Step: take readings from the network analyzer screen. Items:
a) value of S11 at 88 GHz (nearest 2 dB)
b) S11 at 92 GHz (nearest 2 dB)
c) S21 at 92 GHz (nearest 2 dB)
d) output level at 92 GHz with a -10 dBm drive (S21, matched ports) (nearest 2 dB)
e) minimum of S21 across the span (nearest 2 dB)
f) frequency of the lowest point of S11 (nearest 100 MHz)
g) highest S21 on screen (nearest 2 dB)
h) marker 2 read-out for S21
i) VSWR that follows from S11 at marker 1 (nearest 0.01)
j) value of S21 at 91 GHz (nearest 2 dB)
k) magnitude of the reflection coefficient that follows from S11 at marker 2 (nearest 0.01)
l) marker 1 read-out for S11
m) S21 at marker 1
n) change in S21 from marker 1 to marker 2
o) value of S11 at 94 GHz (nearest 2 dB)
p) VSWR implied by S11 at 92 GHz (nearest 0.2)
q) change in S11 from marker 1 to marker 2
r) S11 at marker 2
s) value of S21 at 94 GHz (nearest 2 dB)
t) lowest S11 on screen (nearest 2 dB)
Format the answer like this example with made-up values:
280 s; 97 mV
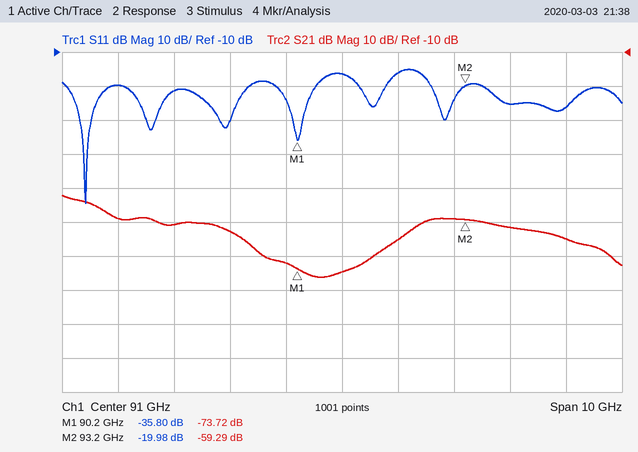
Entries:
-22 dB; -16 dB; -66 dB; -76 dBm; -76 dB; 86.4 GHz; -52 dB; -59.29 dB; 1.03; -74 dB; 0.10; -35.80 dB; -73.72 dB; 14.43 dB; -26 dB; 1.4; 15.82 dB; -19.98 dB; -62 dB; -54 dB
